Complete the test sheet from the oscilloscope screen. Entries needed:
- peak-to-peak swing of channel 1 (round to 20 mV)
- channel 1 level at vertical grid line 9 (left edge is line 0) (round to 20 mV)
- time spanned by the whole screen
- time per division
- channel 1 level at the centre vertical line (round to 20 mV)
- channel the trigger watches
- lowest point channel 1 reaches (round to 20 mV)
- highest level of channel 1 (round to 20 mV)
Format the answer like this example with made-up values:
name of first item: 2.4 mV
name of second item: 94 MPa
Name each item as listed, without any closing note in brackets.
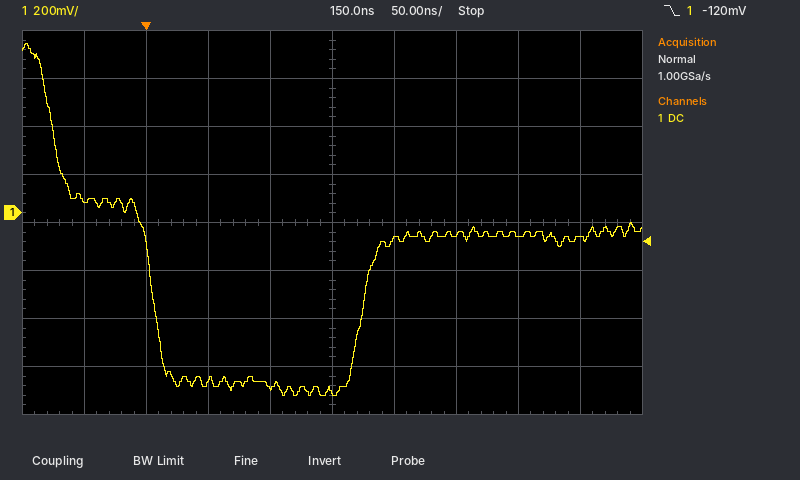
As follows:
peak-to-peak swing of channel 1: 1.46 V
channel 1 level at vertical grid line 9 (left edge is line 0): -100 mV
time spanned by the whole screen: 500 ns
time per division: 50 ns
channel 1 level at the centre vertical line: -740 mV
channel the trigger watches: channel 1
lowest point channel 1 reaches: -760 mV
highest level of channel 1: 700 mV
